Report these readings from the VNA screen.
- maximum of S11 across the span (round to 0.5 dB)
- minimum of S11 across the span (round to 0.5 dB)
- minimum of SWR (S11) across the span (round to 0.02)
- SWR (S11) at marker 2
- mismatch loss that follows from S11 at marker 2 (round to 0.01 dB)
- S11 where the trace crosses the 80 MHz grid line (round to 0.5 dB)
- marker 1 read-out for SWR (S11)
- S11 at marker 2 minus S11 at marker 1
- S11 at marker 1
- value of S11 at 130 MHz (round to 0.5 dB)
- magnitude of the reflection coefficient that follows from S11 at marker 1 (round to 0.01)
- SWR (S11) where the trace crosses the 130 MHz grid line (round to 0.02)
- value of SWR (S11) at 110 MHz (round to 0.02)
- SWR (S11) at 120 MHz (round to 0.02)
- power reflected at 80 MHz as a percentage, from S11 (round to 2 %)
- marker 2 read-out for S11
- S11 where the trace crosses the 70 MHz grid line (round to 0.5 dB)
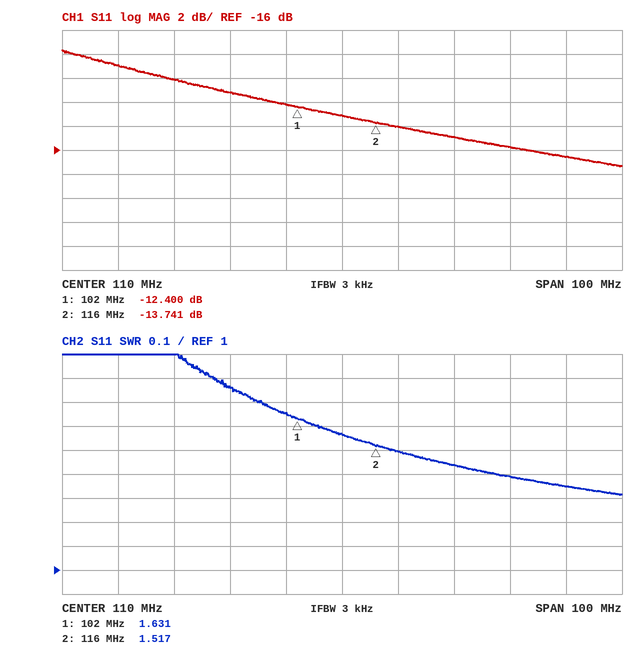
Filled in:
-7.5 dB
-17.5 dB
1.32
1.517
0.19 dB
-10.0 dB
1.631
-1.341 dB
-12.400 dB
-15.0 dB
0.24
1.44
1.56
1.50
10 %
-13.741 dB
-9.0 dB
